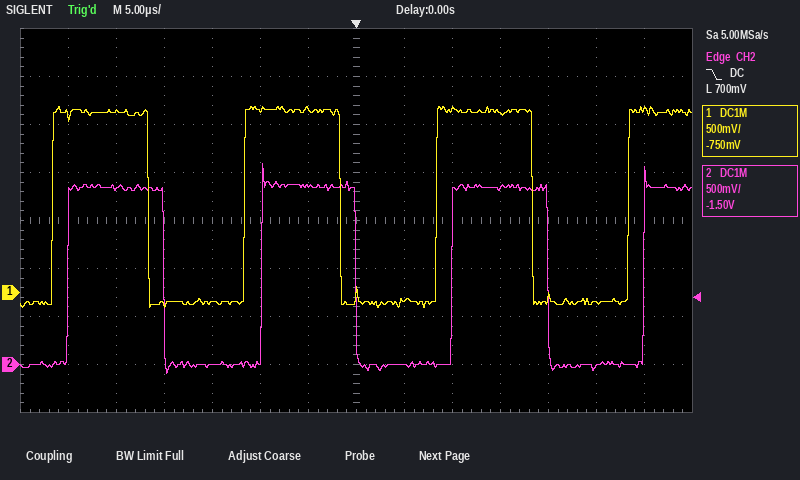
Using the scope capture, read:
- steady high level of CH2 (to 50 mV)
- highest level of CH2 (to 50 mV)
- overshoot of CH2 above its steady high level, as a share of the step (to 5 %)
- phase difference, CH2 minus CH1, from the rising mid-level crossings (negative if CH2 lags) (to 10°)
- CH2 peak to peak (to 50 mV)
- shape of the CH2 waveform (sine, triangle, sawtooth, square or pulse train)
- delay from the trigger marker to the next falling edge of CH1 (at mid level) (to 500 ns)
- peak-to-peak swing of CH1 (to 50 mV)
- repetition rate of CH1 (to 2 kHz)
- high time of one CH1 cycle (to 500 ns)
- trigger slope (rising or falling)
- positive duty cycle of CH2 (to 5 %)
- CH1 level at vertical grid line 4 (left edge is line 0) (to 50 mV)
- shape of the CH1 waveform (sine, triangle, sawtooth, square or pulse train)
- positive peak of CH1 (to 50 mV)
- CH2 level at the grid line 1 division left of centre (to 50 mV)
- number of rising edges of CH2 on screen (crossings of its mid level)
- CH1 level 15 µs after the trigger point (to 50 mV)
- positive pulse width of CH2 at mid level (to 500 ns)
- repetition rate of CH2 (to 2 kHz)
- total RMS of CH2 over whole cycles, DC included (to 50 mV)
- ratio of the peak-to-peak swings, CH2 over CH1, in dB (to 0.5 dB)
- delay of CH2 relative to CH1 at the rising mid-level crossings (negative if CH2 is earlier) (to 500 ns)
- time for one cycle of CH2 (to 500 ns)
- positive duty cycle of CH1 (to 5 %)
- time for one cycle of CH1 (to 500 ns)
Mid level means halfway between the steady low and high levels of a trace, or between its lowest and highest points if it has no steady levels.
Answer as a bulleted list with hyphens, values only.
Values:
- 1.85 V
- 2.10 V
- 15 %
- -30°
- 2.20 V
- square
- 18.5 µs
- 2.10 V
- 50 kHz
- 10.0 µs
- falling
- 50 %
- -100 mV
- square
- 1.95 V
- 1.85 V
- 4
- 1.85 V
- 10.0 µs
- 50 kHz
- 1.30 V
- 0.5 dB
- +1.5 µs
- 20.0 µs
- 50 %
- 20.0 µs
